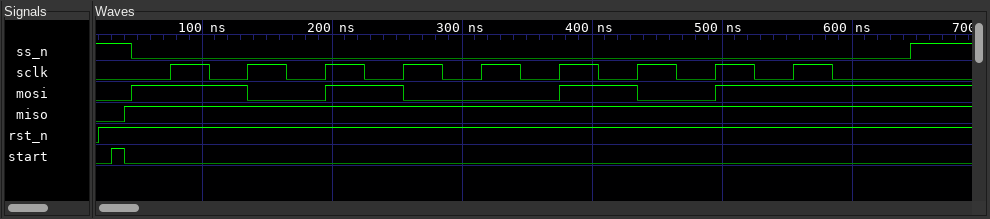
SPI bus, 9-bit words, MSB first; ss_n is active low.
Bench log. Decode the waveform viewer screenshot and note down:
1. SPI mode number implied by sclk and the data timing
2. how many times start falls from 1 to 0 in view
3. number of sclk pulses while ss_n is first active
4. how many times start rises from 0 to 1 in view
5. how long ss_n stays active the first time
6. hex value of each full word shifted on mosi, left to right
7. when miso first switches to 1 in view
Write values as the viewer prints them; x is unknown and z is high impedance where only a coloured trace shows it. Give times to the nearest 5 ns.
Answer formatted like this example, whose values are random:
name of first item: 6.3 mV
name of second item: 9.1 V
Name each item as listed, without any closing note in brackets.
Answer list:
SPI mode number implied by sclk and the data timing: 1
how many times start falls from 1 to 0 in view: 1
number of sclk pulses while ss_n is first active: 9
how many times start rises from 0 to 1 in view: 1
how long ss_n stays active the first time: 600 ns
hex value of each full word shifted on mosi, left to right: 14B
when miso first switches to 1 in view: 40 ns
